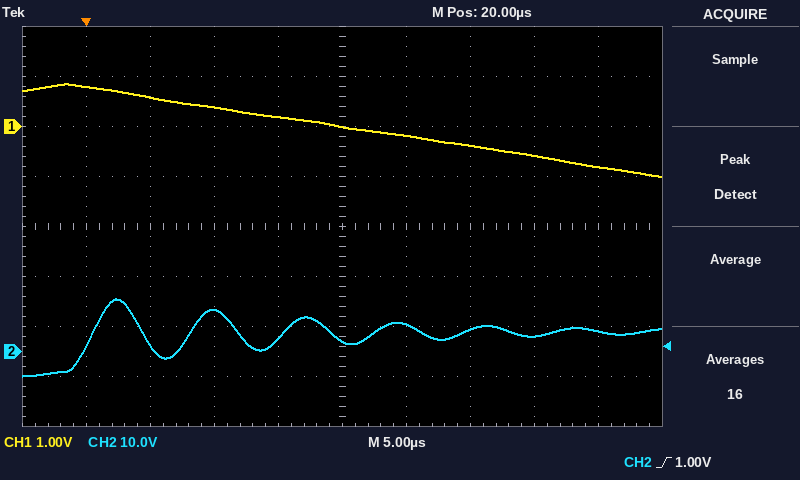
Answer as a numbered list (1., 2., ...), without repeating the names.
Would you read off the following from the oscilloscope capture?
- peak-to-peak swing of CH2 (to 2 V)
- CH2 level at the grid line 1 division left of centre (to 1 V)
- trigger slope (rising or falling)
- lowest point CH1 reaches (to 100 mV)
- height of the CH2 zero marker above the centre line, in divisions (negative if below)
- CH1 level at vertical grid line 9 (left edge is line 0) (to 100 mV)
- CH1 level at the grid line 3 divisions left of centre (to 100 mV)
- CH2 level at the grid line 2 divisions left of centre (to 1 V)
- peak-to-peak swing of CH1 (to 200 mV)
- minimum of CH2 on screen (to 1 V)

1. 16 V
2. 3 V
3. rising
4. -1.0 V
5. -2.5 div
6. -800 mV
7. 600 mV
8. 8 V
9. 1.8 V
10. -5 V
